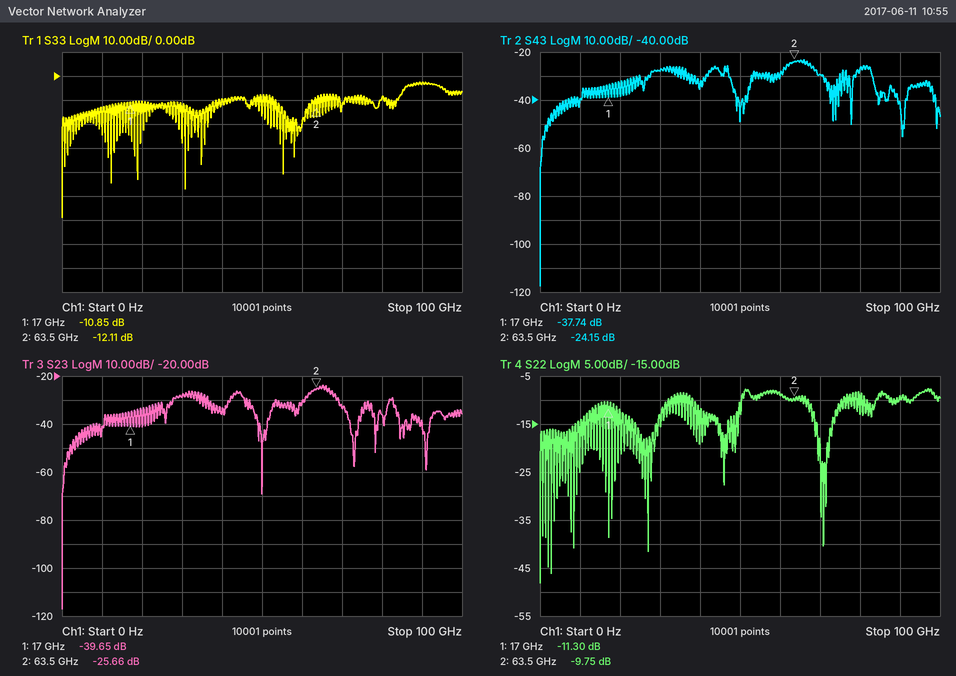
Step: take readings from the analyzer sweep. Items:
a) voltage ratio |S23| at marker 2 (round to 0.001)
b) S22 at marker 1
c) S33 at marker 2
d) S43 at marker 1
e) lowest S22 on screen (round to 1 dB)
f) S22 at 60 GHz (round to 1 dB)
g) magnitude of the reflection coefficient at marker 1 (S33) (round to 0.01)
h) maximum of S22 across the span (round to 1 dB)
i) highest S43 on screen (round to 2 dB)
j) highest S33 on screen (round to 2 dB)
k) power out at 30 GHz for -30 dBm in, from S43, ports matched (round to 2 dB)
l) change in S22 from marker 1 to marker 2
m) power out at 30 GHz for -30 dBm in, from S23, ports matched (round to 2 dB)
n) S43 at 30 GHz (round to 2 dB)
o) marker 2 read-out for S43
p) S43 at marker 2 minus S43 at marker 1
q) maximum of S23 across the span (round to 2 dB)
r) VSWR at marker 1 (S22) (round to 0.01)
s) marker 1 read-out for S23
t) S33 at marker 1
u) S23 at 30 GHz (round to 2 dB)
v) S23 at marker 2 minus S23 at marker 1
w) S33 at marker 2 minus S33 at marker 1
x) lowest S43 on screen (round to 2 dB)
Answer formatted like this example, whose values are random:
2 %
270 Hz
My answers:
0.052
-11.30 dB
-12.11 dB
-37.74 dB
-48 dB
-9 dB
0.29
-8 dB
-24 dB
-2 dB
-58 dBm
1.55 dB
-58 dBm
-28 dB
-24.15 dB
13.59 dB
-24 dB
1.75
-39.65 dB
-10.85 dB
-28 dB
13.99 dB
-1.26 dB
-118 dB
